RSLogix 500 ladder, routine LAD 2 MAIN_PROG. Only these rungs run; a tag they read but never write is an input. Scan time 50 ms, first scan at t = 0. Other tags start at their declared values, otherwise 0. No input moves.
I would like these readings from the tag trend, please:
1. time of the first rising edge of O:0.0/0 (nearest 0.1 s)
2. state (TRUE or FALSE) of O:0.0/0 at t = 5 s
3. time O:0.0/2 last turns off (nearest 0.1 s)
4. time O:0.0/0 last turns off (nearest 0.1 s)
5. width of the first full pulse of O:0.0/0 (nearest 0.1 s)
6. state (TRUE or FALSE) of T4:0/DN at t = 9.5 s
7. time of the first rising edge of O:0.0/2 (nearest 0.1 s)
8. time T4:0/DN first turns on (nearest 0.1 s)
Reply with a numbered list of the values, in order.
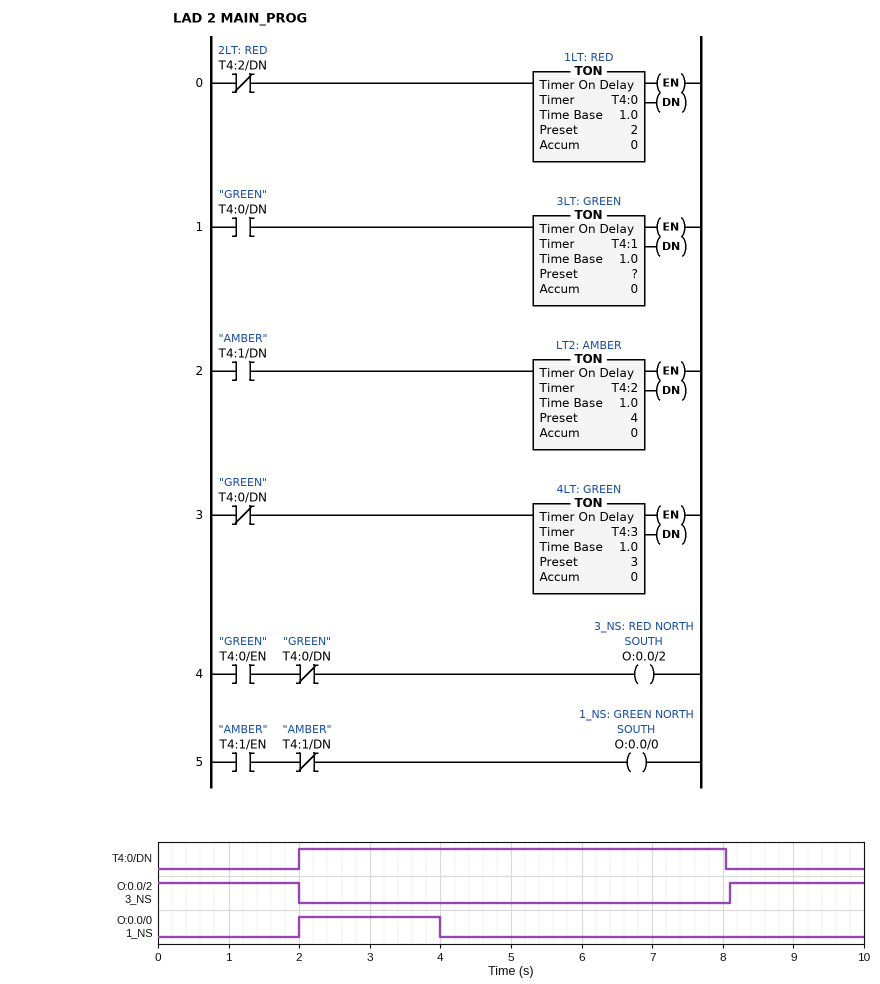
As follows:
1. 2.0 s
2. FALSE
3. 2.0 s
4. 4.0 s
5. 2.0 s
6. FALSE
7. 8.1 s
8. 2.0 s
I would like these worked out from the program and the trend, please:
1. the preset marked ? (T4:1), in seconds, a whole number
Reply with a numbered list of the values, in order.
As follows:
1. 2 s
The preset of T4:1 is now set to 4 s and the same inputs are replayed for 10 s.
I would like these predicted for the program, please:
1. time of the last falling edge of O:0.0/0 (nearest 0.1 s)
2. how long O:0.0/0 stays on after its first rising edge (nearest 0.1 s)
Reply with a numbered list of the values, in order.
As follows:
1. 6.0 s
2. 4.0 s
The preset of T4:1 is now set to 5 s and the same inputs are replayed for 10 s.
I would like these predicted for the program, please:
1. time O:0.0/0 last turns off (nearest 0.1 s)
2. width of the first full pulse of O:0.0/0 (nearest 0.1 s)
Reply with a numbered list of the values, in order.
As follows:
1. 7.0 s
2. 5.0 s
